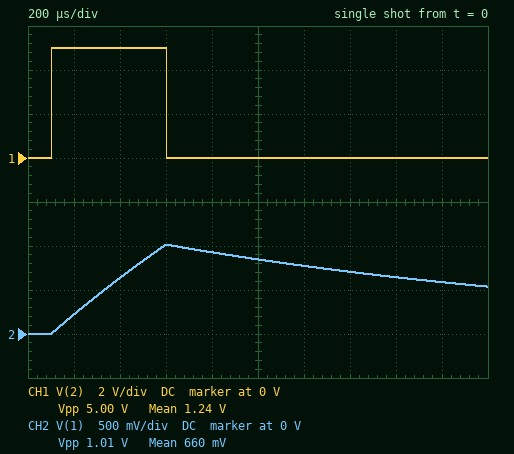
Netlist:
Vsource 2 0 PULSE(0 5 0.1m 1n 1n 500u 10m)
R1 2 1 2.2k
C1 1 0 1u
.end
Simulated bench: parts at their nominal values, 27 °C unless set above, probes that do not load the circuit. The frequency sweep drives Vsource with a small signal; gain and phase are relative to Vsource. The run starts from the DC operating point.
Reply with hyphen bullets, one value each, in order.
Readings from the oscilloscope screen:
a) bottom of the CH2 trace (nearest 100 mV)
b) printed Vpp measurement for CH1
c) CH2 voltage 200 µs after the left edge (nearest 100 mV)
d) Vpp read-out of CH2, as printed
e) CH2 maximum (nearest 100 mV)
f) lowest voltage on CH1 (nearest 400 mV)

- 0 V
- 5.00 V
- 200 mV
- 1.01 V
- 1.0 V
- 0 V
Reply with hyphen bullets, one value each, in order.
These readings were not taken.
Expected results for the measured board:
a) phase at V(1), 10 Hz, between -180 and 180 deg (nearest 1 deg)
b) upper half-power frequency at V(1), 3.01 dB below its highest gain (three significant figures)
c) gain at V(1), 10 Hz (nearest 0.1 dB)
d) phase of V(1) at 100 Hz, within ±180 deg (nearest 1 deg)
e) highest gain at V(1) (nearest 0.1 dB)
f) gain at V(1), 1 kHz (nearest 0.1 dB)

- -8 deg
- 72.3 Hz
- -0.1 dB
- -54 deg
- 0 dB
- -22.8 dB
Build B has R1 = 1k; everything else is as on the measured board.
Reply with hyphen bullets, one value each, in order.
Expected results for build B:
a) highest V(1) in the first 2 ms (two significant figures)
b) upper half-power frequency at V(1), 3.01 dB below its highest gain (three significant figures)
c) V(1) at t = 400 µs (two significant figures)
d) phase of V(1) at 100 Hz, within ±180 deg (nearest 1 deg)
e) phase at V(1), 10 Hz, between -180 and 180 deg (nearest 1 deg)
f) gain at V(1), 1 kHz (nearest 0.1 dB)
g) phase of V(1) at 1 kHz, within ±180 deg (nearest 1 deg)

- 2.0 V
- 159 Hz
- 1.3 V
- -32 deg
- -4 deg
- -16.1 dB
- -81 deg
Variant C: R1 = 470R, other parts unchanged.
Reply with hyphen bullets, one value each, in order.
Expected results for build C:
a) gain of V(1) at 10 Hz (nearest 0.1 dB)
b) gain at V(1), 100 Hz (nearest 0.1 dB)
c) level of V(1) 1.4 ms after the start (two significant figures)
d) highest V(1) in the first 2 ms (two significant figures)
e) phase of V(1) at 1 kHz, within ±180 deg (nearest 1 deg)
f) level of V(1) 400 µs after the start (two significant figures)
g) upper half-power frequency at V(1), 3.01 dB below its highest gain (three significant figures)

- 0 dB
- -0.4 dB
- 600 mV
- 3.3 V
- -71 deg
- 2.4 V
- 339 Hz
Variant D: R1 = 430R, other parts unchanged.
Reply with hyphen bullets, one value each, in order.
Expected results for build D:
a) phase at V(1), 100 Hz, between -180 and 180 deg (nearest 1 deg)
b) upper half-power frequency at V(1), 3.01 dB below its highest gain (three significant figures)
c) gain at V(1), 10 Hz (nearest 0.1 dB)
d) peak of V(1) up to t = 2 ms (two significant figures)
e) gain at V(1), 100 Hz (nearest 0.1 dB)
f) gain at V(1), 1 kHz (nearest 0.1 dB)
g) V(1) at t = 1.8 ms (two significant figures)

- -15 deg
- 370 Hz
- 0 dB
- 3.4 V
- -0.3 dB
- -9.2 dB
- 210 mV
